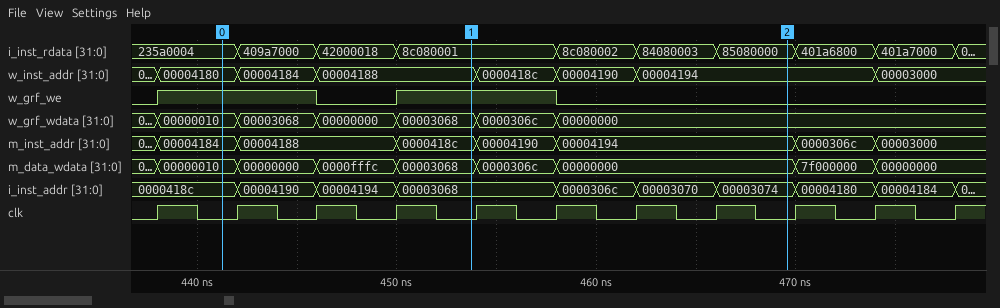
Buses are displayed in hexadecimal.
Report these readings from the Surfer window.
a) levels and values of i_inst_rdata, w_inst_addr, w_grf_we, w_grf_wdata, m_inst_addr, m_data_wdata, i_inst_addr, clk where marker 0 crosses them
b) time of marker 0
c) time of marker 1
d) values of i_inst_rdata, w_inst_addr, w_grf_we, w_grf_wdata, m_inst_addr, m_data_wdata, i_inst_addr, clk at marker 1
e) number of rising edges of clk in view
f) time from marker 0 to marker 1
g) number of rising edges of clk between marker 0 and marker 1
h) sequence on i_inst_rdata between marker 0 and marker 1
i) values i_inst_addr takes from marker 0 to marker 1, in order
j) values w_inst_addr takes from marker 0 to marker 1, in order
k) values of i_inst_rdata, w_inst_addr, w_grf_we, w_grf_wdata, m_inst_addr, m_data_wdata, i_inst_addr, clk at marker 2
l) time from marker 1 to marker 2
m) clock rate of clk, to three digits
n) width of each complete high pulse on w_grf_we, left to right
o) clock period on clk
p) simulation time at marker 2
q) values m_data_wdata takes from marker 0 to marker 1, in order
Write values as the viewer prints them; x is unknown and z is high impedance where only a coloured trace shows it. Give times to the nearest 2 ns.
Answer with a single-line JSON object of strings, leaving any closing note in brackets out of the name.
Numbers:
{"levels and values of i_inst_rdata, w_inst_addr, w_grf_we, w_grf_wdata, m_inst_addr, m_data_wdata, i_inst_addr, clk where marker 0 crosses them": "i_inst_rdata=235a0004, w_inst_addr=00004180, w_grf_we=1, w_grf_wdata=00000010, m_inst_addr=00004184, m_data_wdata=00000010, i_inst_addr=0000418c, clk=0", "time of marker 0": "442 ns", "time of marker 1": "454 ns", "values of i_inst_rdata, w_inst_addr, w_grf_we, w_grf_wdata, m_inst_addr, m_data_wdata, i_inst_addr, clk at marker 1": "i_inst_rdata=8c080001, w_inst_addr=00004188, w_grf_we=1, w_grf_wdata=00003068, m_inst_addr=0000418c, m_data_wdata=00003068, i_inst_addr=00003068, clk=0", "number of rising edges of clk in view": "11", "time from marker 0 to marker 1": "12 ns", "number of rising edges of clk between marker 0 and marker 1": "3", "sequence on i_inst_rdata between marker 0 and marker 1": "235a0004, 409a7000, 42000018, 8c080001", "values i_inst_addr takes from marker 0 to marker 1, in order": "0000418c, 00004190, 00004194, 00003068", "values w_inst_addr takes from marker 0 to marker 1, in order": "00004180, 00004184, 00004188", "values of i_inst_rdata, w_inst_addr, w_grf_we, w_grf_wdata, m_inst_addr, m_data_wdata, i_inst_addr, clk at marker 2": "i_inst_rdata=85080000, w_inst_addr=00004194, w_grf_we=0, w_grf_wdata=00000000, m_inst_addr=00004194, m_data_wdata=00000000, i_inst_addr=00003074, clk=0", "time from marker 1 to marker 2": "16 ns", "clock rate of clk, to three digits": "250 MHz", "width of each complete high pulse on w_grf_we, left to right": "8 ns, 8 ns", "clock period on clk": "4 ns", "simulation time at marker 2": "470 ns", "values m_data_wdata takes from marker 0 to marker 1, in order": "00000010, 00000000, 0000fffc, 00003068"}
